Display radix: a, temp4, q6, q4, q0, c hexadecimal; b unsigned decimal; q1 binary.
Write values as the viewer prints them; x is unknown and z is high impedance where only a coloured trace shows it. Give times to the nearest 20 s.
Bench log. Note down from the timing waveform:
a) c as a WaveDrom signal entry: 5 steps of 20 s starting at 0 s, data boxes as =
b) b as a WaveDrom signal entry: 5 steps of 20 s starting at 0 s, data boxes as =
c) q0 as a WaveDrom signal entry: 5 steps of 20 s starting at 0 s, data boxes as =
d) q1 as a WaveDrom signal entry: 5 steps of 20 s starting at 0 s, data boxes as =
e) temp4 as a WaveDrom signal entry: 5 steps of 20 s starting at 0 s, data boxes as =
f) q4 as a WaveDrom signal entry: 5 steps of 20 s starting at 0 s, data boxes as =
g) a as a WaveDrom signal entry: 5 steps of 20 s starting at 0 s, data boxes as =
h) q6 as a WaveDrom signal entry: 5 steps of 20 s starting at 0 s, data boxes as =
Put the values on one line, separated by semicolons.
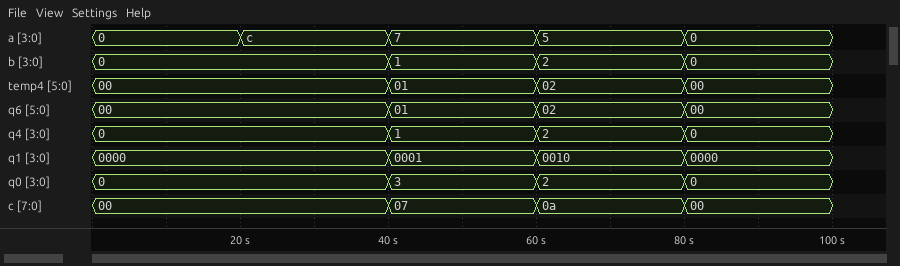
{name: 'c', wave: '=.===', data: '00 07 0a 00'}; {name: 'b', wave: '=.===', data: '0 1 2 0'}; {name: 'q0', wave: '=.===', data: '0 3 2 0'}; {name: 'q1', wave: '=.===', data: '0000 0001 0010 0000'}; {name: 'temp4', wave: '=.===', data: '00 01 02 00'}; {name: 'q4', wave: '=.===', data: '0 1 2 0'}; {name: 'a', wave: '=====', data: '0 c 7 5 0'}; {name: 'q6', wave: '=.===', data: '00 01 02 00'}
